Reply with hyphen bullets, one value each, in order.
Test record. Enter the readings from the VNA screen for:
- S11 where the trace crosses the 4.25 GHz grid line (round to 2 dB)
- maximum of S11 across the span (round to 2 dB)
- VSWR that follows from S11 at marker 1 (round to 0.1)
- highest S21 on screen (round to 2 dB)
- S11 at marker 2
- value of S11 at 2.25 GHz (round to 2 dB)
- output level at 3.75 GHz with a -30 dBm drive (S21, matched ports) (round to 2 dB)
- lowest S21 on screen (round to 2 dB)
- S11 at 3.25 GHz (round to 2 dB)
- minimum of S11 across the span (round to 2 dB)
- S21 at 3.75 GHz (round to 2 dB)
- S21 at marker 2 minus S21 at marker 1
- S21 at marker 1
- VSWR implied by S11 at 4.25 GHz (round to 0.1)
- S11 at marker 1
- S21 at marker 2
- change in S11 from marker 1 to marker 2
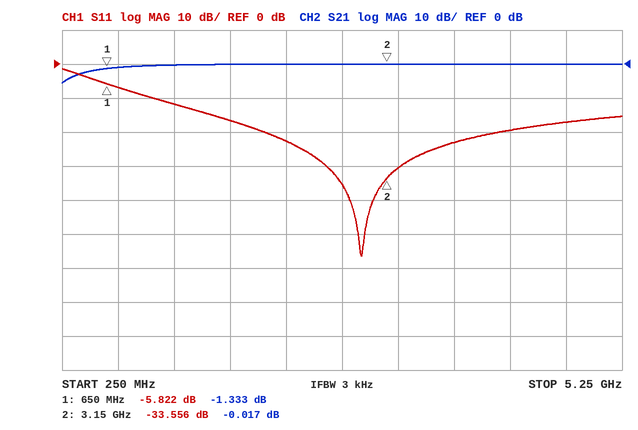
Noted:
- -20 dB
- -2 dB
- 3.1
- 0 dB
- -33.556 dB
- -22 dB
- -30 dBm
- -6 dB
- -30 dB
- -56 dB
- 0 dB
- 1.316 dB
- -1.333 dB
- 1.2
- -5.822 dB
- -0.017 dB
- -27.734 dB
